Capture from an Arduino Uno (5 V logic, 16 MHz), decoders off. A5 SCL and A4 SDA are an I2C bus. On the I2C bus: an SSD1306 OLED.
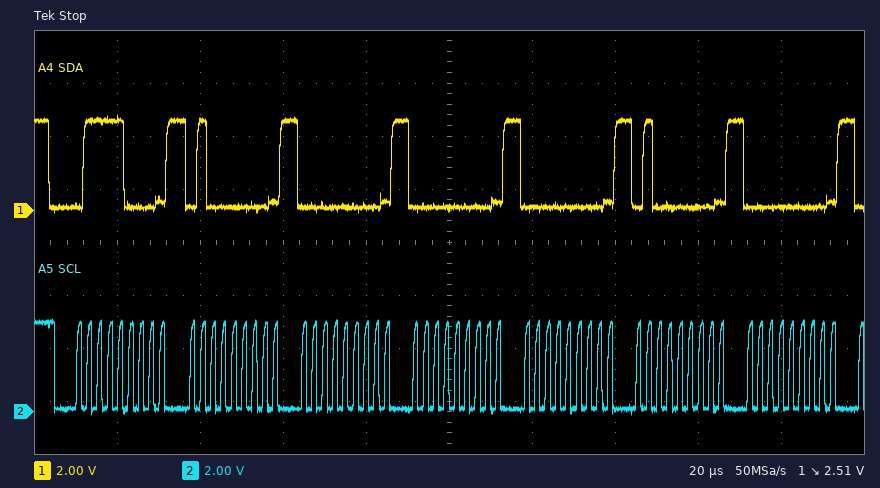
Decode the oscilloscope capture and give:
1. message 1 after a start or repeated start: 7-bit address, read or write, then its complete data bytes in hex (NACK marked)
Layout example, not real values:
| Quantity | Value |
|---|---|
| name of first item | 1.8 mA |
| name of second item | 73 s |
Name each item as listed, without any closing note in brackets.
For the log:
| Quantity | Value |
|---|---|
| message 1 after a start or repeated start: 7-bit address, read or write, then its complete data bytes in hex | 0x3C write: 40 00 00 00 40 00 |
